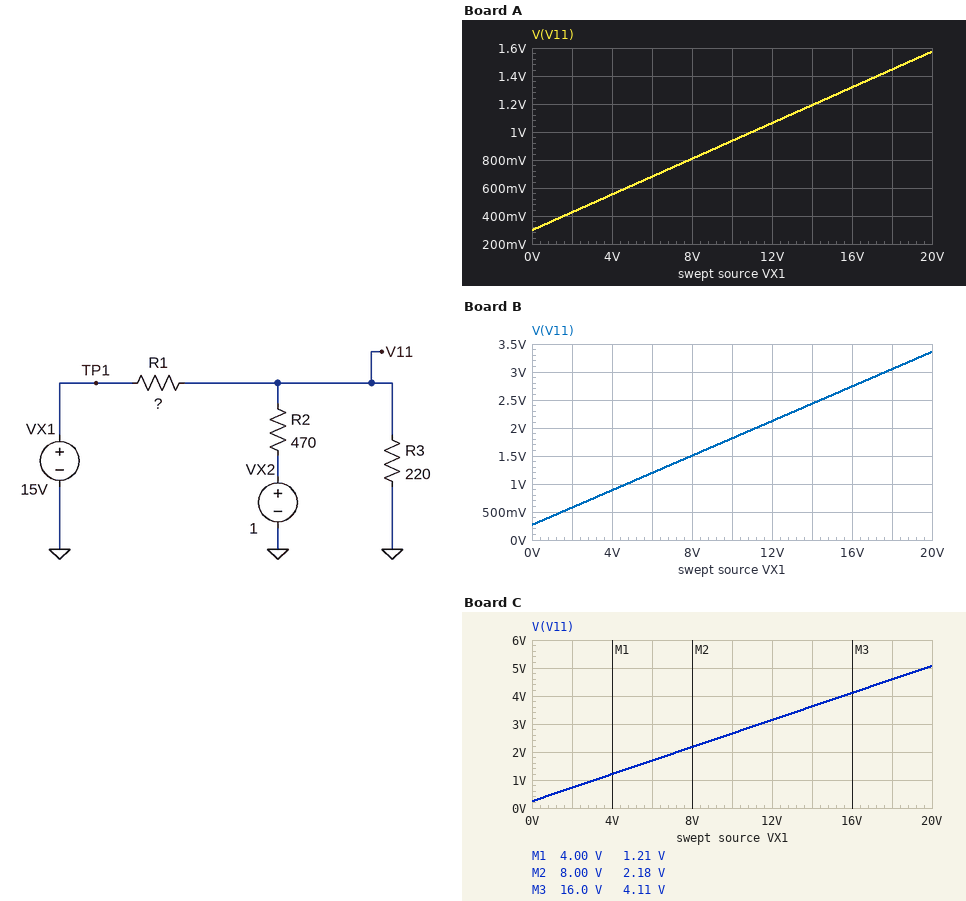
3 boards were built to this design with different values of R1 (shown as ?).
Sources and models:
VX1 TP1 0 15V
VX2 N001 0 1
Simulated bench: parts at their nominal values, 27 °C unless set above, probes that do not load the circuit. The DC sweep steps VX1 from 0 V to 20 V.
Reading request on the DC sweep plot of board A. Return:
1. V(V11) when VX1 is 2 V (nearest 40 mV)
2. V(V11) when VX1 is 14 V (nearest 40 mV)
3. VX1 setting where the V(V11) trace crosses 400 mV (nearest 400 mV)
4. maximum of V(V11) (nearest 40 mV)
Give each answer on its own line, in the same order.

440 mV
1.20 V
1.6 V
1.56 V
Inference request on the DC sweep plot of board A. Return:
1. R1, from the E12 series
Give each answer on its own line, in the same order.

2.2 kΩ
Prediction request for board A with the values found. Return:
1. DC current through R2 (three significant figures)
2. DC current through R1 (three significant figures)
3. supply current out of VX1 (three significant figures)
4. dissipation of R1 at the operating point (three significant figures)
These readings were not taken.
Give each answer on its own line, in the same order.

543 µA
6.25 mA
6.25 mA
85.9 mW
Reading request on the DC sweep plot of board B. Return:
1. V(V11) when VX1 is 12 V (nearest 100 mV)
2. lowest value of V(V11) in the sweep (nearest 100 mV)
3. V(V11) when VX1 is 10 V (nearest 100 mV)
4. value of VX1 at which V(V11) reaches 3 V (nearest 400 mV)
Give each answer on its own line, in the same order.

2.1 V
300 mV
1.8 V
17.6 V
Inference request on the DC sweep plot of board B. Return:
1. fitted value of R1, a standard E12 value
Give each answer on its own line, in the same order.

820 Ω
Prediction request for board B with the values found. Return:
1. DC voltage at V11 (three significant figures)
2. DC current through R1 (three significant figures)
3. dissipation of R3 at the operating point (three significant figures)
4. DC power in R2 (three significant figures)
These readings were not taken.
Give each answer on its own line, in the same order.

2.59 V
15.1 mA
30.4 mW
5.36 mW
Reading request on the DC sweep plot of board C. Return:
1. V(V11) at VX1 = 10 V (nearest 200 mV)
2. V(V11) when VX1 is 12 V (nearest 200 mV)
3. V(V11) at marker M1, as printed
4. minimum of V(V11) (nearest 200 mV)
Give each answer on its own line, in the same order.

2.6 V
3.2 V
1.21 V
200 mV
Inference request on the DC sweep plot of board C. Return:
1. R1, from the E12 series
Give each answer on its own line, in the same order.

470 Ω
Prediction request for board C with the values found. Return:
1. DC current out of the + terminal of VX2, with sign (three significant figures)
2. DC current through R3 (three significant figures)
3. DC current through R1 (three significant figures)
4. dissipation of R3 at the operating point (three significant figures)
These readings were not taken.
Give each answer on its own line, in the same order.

-6.10 mA
17.6 mA
23.7 mA
68.0 mW
